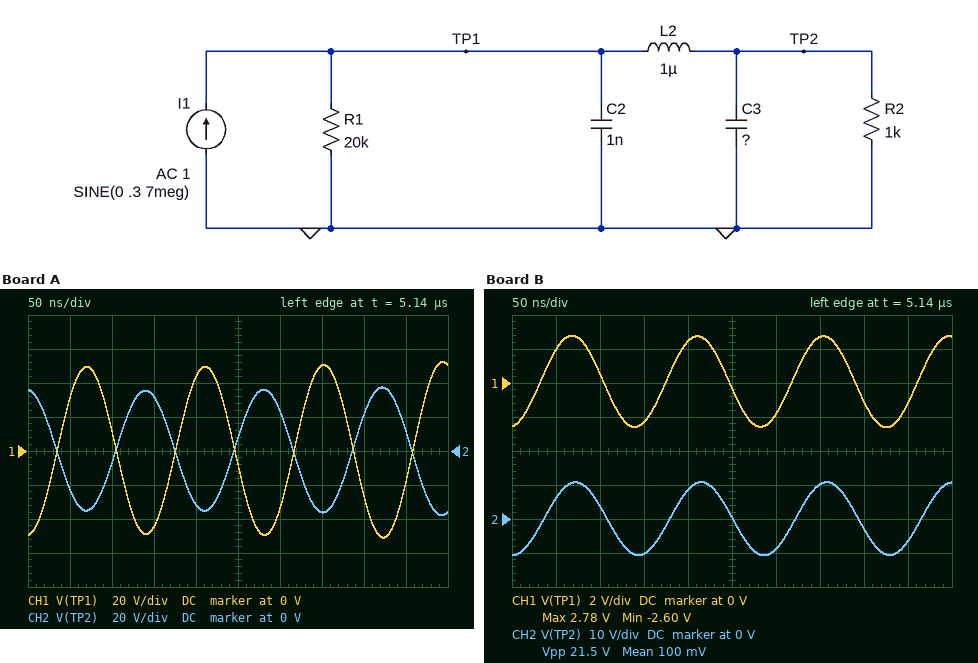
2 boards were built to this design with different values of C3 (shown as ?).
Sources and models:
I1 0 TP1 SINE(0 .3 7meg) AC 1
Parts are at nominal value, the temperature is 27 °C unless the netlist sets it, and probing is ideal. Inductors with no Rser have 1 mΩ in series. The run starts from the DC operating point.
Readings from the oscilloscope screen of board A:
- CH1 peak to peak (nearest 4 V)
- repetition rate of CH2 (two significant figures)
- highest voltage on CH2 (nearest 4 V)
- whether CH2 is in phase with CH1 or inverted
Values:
104 V
7.1 MHz
36 V
inverted
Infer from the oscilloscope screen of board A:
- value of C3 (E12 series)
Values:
1.2 nF
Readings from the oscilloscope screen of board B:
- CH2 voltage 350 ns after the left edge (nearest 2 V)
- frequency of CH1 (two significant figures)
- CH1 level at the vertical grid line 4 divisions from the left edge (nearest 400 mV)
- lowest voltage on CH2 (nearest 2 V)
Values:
10 V
7.0 MHz
2.4 V
-10 V
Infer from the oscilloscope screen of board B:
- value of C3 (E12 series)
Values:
390 pF
